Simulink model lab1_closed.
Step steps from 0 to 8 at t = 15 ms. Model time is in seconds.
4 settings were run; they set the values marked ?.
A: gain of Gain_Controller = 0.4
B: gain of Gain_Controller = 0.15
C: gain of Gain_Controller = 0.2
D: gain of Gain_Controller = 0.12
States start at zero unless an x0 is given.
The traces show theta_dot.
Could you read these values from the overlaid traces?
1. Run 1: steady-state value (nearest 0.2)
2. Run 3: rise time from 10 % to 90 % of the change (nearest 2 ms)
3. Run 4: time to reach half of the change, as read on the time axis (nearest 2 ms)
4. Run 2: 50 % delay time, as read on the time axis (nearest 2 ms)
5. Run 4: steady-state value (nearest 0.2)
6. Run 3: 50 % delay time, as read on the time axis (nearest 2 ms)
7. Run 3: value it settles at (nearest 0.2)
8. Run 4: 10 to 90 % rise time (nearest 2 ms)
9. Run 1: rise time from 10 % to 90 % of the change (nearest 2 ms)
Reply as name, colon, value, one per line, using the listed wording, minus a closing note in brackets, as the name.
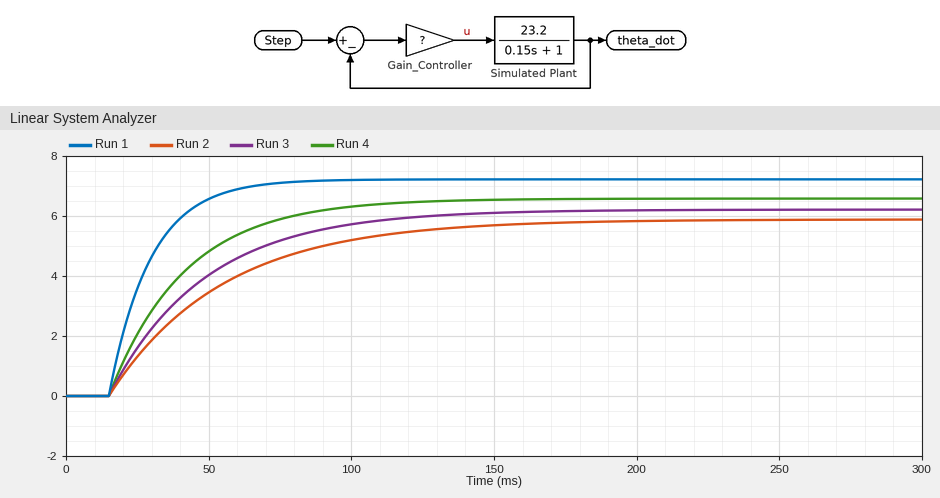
Run 1: steady-state value: 7.2
Run 3: rise time from 10 % to 90 % of the change: 74 ms
Run 4: time to reach half of the change, as read on the time axis: 34 ms
Run 2: 50 % delay time, as read on the time axis: 42 ms
Run 4: steady-state value: 6.6
Run 3: 50 % delay time, as read on the time axis: 38 ms
Run 3: value it settles at: 6.2
Run 4: 10 to 90 % rise time: 58 ms
Run 1: rise time from 10 % to 90 % of the change: 32 ms
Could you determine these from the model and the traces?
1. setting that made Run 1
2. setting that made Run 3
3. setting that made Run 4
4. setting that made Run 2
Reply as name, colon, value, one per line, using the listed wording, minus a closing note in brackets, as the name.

setting that made Run 1: A
setting that made Run 3: B
setting that made Run 4: C
setting that made Run 2: D
